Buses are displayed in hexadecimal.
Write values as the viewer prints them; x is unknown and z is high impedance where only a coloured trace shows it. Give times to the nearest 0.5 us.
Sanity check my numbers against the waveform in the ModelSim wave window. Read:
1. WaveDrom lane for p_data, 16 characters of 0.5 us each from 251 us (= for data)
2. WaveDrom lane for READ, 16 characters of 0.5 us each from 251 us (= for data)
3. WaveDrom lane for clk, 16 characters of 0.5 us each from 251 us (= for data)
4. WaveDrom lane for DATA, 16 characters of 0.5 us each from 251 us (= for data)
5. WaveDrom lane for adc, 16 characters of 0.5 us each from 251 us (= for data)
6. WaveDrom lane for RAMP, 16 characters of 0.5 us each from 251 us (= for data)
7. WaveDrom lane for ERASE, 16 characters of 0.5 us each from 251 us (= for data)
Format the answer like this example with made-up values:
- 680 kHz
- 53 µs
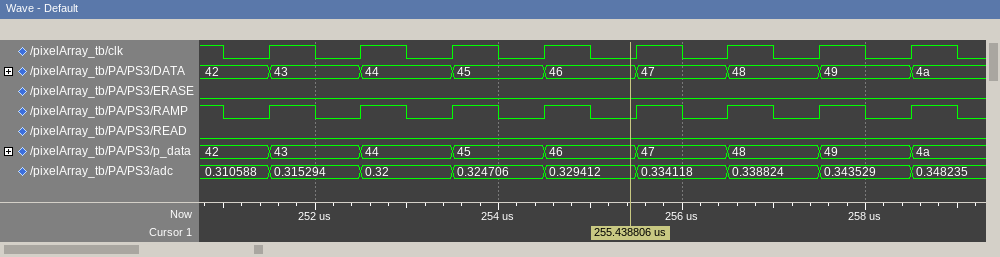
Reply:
- {name: 'p_data', wave: '==.=.=.=.=.=.=.=', data: '42 43 44 45 46 47 48 49 4a'}
- {name: 'READ', wave: '0...............'}
- {name: 'clk', wave: '0101010101010101'}
- {name: 'DATA', wave: '==.=.=.=.=.=.=.=', data: '42 43 44 45 46 47 48 49 4a'}
- {name: 'adc', wave: '==.=.=.=.=.=.=.=', data: '0.310588 0.315294 0.32 0.324706 0.329412 0.334118 0.338824 0.343529 0.348235'}
- {name: 'RAMP', wave: '0101010101010101'}
- {name: 'ERASE', wave: '0...............'}
